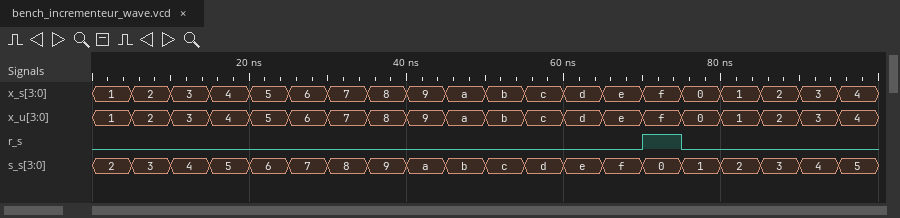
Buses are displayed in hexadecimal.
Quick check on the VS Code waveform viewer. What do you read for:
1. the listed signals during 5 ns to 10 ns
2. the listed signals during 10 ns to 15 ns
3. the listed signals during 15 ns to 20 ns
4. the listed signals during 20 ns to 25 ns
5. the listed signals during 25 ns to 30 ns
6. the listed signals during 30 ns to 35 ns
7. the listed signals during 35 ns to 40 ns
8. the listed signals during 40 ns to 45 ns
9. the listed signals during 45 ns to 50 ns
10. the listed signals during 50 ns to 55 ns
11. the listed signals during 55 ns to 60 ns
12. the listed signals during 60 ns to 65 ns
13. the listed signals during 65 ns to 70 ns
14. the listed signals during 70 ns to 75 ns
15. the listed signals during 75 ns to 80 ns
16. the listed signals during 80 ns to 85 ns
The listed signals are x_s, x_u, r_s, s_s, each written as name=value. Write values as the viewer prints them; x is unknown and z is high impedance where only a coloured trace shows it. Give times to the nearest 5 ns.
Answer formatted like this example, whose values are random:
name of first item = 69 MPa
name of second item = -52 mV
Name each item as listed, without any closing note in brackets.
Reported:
the listed signals during 5 ns to 10 ns = x_s=2, x_u=2, r_s=0, s_s=3
the listed signals during 10 ns to 15 ns = x_s=3, x_u=3, r_s=0, s_s=4
the listed signals during 15 ns to 20 ns = x_s=4, x_u=4, r_s=0, s_s=5
the listed signals during 20 ns to 25 ns = x_s=5, x_u=5, r_s=0, s_s=6
the listed signals during 25 ns to 30 ns = x_s=6, x_u=6, r_s=0, s_s=7
the listed signals during 30 ns to 35 ns = x_s=7, x_u=7, r_s=0, s_s=8
the listed signals during 35 ns to 40 ns = x_s=8, x_u=8, r_s=0, s_s=9
the listed signals during 40 ns to 45 ns = x_s=9, x_u=9, r_s=0, s_s=a
the listed signals during 45 ns to 50 ns = x_s=a, x_u=a, r_s=0, s_s=b
the listed signals during 50 ns to 55 ns = x_s=b, x_u=b, r_s=0, s_s=c
the listed signals during 55 ns to 60 ns = x_s=c, x_u=c, r_s=0, s_s=d
the listed signals during 60 ns to 65 ns = x_s=d, x_u=d, r_s=0, s_s=e
the listed signals during 65 ns to 70 ns = x_s=e, x_u=e, r_s=0, s_s=f
the listed signals during 70 ns to 75 ns = x_s=f, x_u=f, r_s=1, s_s=0
the listed signals during 75 ns to 80 ns = x_s=0, x_u=0, r_s=0, s_s=1
the listed signals during 80 ns to 85 ns = x_s=1, x_u=1, r_s=0, s_s=2
